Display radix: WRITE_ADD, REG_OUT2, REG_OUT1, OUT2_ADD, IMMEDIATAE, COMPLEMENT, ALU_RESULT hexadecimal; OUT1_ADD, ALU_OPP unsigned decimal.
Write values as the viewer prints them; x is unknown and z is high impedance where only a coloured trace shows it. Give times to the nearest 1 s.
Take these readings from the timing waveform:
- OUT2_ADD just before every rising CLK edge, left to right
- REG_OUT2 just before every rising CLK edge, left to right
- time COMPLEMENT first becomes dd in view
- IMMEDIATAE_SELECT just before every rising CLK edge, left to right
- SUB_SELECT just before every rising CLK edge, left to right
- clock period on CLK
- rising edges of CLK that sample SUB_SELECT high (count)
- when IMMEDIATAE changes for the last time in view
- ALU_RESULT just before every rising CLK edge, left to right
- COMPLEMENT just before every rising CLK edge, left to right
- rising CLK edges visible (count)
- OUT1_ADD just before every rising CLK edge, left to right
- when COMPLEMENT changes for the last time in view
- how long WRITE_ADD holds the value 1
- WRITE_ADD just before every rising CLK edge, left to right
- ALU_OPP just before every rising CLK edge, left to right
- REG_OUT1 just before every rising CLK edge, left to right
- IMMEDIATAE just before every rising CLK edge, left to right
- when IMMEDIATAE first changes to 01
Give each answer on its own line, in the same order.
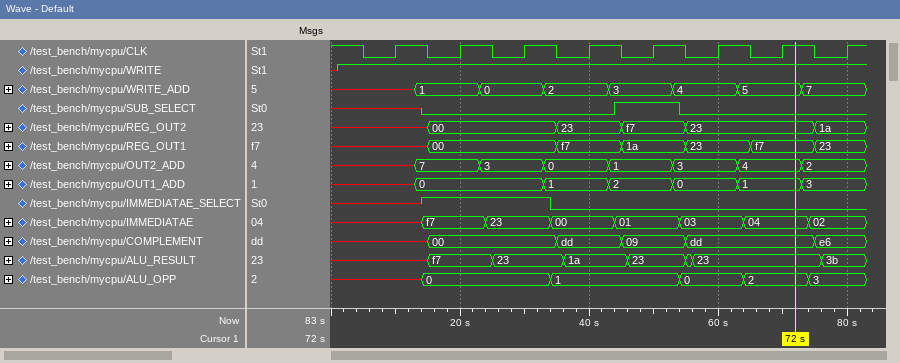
x, 7, 3, 0, 1, 3, 4, 2
x, 00, 00, 23, f7, 23, 23, 1a
35 s
x 1 1 0 0 0 0 0
x 0 0 0 1 0 0 0
10 s
1
74 s
x, f7, 23, 1a, 23, 23, 23, 3b
x, 00, 00, dd, 09, dd, dd, e6
8
x, 0, 0, 1, 2, 0, 1, 3
75 s
10 s
x, 1, 0, 2, 3, 4, 5, 7
x, 0, 0, 1, 1, 0, 2, 3
x, 00, 00, f7, 1a, 23, f7, 23
x, f7, 23, 00, 01, 03, 04, 02
44 s
